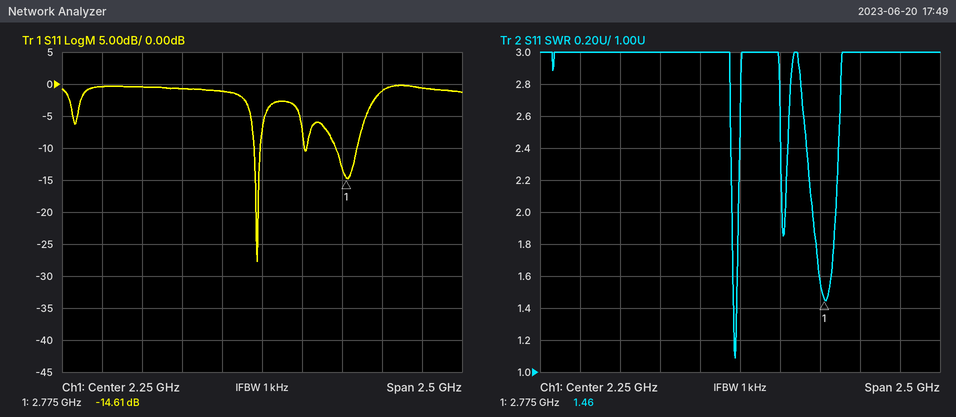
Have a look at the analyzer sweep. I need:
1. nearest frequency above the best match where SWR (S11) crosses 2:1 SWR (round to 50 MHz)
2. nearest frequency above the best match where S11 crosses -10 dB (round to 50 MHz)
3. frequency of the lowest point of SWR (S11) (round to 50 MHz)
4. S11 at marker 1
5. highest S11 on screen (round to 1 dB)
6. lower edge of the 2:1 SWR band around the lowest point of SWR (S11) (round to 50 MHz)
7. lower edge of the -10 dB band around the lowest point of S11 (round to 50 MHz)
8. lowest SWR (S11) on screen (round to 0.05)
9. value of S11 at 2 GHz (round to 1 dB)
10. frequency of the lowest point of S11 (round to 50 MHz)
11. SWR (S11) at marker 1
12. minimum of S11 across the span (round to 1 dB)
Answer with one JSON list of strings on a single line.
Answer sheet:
["2.25 GHz", "2.25 GHz", "2.20 GHz", "-14.61 dB", "0 dB", "2.20 GHz", "2.20 GHz", "1.10", "-1 dB", "2.20 GHz", "1.46", "-28 dB"]
